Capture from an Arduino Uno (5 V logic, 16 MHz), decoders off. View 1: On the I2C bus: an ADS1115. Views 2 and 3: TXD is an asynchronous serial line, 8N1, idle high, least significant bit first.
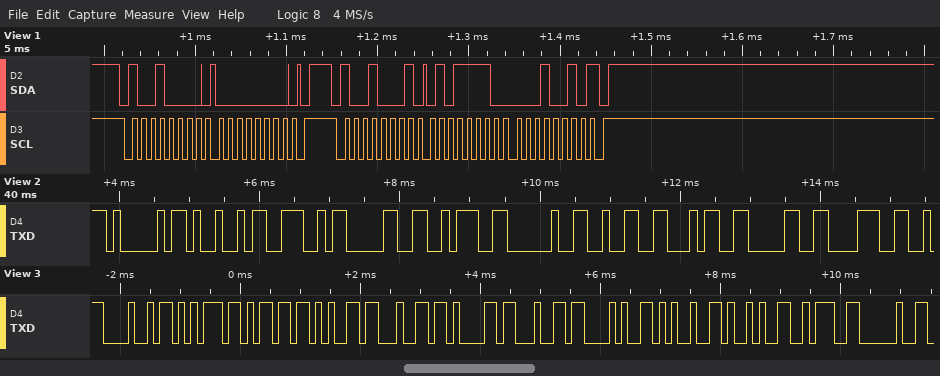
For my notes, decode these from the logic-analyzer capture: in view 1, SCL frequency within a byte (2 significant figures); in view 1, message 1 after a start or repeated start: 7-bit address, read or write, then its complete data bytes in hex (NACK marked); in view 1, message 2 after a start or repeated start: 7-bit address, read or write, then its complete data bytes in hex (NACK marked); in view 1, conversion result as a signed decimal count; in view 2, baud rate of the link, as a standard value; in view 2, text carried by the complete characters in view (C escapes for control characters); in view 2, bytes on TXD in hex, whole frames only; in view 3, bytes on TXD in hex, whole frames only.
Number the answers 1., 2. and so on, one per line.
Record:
1. 100 kHz
2. 0x48 write: 00
3. 0x48 read: 5E 12 NACK
4. 24082
5. 9600 baud
6. "AIN0: 2408"
7. 0x41 0x49 0x4E 0x30 0x3A 0x20 0x32 0x34 0x30 0x38
8. 48 75 6D 65 64 61 64 28 25 29 3A 20
